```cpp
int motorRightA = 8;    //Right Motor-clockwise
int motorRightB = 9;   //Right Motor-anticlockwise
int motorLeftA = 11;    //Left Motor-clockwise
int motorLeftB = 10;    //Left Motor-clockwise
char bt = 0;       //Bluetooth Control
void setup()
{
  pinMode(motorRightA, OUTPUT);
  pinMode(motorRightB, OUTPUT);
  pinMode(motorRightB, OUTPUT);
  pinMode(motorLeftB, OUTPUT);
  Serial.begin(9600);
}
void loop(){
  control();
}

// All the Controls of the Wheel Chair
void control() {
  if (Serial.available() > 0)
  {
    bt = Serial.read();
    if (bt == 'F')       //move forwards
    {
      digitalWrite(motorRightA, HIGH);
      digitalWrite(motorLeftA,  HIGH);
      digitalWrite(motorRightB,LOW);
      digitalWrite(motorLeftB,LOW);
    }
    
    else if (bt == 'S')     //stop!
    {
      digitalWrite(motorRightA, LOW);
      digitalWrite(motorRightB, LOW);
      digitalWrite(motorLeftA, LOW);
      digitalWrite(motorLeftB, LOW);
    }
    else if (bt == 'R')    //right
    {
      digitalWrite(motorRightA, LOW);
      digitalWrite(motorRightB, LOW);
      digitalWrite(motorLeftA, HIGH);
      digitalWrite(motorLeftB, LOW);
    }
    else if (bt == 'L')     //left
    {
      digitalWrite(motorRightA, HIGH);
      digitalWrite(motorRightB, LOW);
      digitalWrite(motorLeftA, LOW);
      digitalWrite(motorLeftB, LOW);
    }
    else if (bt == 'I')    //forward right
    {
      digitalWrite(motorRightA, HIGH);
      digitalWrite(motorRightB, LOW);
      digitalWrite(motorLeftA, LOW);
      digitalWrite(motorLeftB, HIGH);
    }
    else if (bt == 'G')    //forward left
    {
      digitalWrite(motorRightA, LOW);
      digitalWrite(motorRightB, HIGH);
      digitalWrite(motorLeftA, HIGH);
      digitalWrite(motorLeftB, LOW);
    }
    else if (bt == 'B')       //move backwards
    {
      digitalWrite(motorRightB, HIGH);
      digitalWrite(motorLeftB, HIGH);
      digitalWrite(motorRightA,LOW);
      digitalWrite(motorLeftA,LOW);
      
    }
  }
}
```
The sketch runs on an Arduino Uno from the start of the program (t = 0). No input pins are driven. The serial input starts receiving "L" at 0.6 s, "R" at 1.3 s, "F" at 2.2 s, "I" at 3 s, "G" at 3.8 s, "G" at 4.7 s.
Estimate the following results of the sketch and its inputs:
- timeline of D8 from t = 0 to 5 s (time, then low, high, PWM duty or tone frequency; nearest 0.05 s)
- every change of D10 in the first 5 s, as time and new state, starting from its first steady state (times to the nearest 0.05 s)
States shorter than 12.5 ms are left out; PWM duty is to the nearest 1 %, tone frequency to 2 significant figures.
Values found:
0 s low; 0.6 s high; 1.3 s low; 2.2 s high; 3.8 s low
0 s low; 3 s high; 3.8 s low
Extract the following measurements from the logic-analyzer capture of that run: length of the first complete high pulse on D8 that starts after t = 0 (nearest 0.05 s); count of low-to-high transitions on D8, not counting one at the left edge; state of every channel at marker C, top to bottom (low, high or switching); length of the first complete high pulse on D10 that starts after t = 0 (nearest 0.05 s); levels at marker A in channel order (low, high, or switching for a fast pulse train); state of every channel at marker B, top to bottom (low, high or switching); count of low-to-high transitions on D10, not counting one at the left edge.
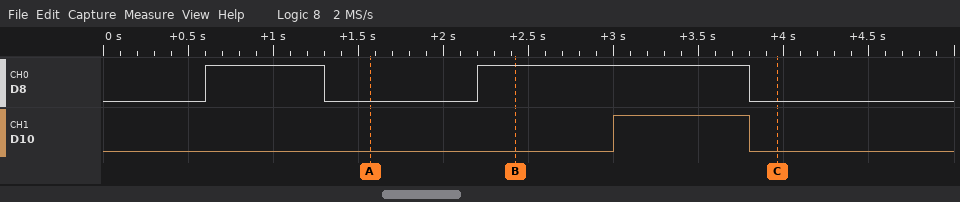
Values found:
0.70 s
2
D8 low, D10 low
0.80 s
D8 low, D10 low
D8 high, D10 low
1
